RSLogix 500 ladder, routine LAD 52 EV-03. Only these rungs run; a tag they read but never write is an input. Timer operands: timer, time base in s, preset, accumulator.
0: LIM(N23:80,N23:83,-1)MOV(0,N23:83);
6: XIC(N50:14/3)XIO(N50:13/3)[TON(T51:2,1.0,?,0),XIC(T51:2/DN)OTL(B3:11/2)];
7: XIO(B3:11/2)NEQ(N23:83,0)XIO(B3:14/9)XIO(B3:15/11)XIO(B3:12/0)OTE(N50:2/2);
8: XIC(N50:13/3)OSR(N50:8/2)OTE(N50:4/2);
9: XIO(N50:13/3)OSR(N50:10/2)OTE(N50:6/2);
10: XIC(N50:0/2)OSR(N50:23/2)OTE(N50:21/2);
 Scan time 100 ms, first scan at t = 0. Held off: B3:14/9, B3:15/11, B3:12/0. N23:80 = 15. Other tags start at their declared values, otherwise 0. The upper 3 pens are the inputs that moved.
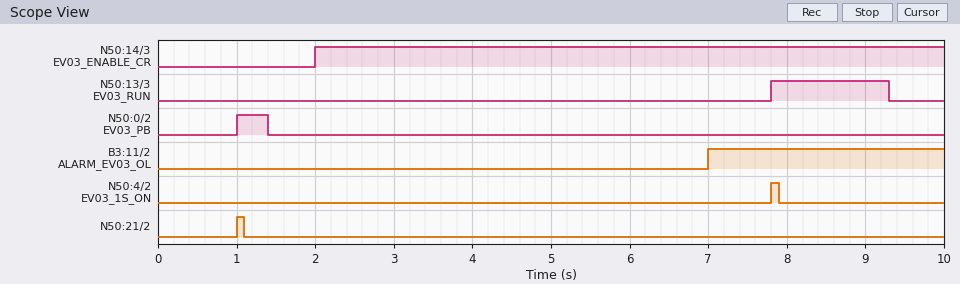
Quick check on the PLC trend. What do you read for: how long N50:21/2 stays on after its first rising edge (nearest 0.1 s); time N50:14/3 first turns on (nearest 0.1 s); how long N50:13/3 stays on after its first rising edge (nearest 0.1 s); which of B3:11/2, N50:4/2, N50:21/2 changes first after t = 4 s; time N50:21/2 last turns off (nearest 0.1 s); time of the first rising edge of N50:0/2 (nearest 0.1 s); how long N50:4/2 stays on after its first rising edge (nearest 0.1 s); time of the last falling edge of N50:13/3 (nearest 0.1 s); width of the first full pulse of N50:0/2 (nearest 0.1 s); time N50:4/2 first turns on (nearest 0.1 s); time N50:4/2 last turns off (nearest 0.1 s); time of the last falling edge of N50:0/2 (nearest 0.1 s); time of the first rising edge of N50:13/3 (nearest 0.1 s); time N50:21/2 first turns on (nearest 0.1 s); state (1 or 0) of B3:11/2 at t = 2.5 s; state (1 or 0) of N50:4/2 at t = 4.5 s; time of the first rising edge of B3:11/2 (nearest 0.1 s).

0.1 s
2.0 s
1.5 s
B3:11/2
1.1 s
1.0 s
0.1 s
9.3 s
0.4 s
7.8 s
7.9 s
1.4 s
7.8 s
1.0 s
0
0
7.0 s
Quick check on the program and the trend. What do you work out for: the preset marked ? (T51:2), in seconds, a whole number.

5 s
